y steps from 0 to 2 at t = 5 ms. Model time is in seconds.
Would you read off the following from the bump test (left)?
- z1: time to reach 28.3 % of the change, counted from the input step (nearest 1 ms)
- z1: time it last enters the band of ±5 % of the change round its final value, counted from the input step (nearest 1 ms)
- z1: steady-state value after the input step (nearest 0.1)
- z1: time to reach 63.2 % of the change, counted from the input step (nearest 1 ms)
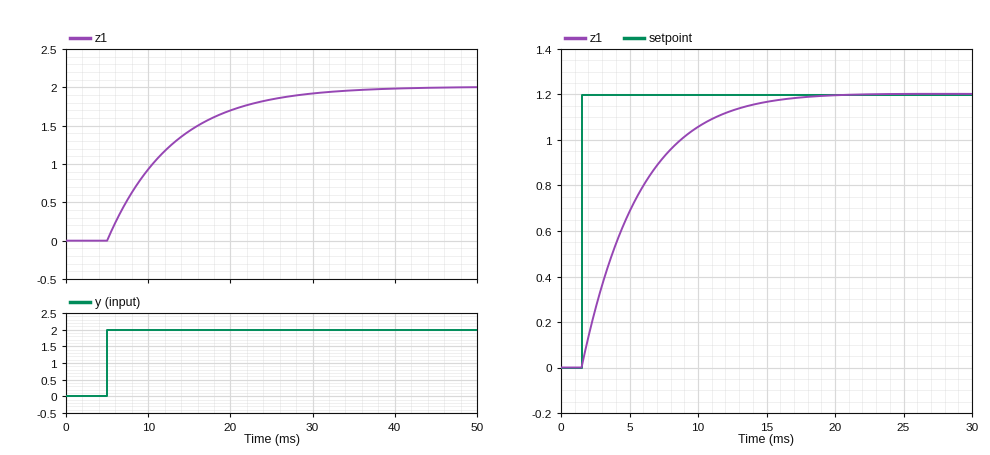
3 ms
24 ms
2.0
8 ms
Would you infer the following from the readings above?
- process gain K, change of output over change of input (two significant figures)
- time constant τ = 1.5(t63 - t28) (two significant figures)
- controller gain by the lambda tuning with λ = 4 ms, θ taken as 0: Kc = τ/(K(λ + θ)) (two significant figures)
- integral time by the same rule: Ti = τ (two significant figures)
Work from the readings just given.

1.0
7.5 ms
1.9
7.5 ms
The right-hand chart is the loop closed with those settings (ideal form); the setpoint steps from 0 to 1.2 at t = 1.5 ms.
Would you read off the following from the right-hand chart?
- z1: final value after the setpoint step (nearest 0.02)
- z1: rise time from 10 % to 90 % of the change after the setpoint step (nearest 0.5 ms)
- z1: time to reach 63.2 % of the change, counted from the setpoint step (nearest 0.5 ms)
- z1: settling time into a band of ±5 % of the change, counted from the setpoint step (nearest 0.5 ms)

1.20
8.5 ms
4.0 ms
11.5 ms
